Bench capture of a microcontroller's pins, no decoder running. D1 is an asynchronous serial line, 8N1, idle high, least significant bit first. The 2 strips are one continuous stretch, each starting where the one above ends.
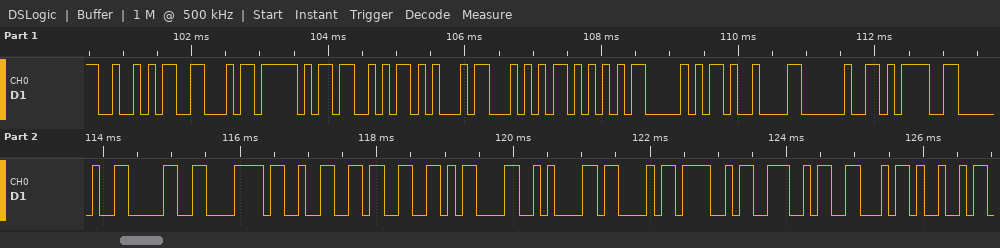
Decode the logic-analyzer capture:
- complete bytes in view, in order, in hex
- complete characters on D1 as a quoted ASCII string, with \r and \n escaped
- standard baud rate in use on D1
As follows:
52 46 5F 53 45 54 55 50 09 20 3D 20 30 78 32 33 0D 0A 43 4F 4E 46 49
"RF_SETUP\t = 0x23\r\nCONFI"
9600 baud
